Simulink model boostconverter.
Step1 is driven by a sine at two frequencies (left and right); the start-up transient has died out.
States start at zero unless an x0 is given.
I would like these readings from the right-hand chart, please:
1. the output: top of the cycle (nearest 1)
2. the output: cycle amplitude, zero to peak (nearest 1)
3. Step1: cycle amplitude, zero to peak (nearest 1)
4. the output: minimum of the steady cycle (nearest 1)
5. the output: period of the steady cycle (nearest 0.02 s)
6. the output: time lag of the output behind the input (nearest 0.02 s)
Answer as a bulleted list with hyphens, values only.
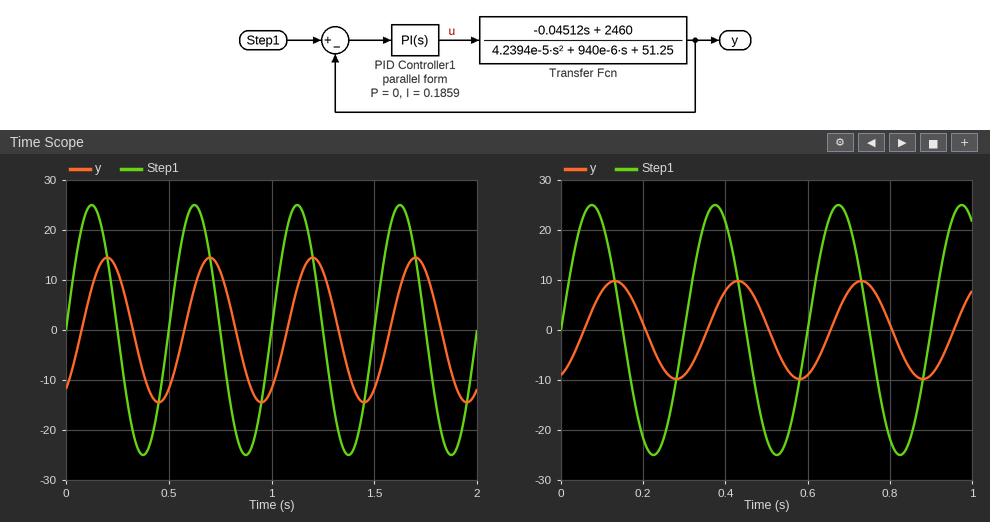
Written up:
- 10
- 10
- 25
- -10
- 0.30 s
- 0.06 s
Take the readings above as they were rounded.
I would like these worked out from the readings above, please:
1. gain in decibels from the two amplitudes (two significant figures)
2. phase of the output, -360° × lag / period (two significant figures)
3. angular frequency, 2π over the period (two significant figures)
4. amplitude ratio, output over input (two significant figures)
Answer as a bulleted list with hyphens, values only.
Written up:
- -8.0 dB
- -72°
- 21 rad/s
- 0.40
